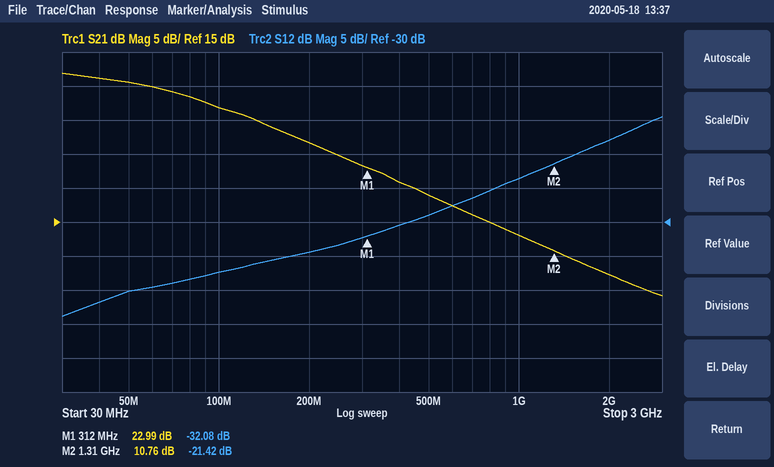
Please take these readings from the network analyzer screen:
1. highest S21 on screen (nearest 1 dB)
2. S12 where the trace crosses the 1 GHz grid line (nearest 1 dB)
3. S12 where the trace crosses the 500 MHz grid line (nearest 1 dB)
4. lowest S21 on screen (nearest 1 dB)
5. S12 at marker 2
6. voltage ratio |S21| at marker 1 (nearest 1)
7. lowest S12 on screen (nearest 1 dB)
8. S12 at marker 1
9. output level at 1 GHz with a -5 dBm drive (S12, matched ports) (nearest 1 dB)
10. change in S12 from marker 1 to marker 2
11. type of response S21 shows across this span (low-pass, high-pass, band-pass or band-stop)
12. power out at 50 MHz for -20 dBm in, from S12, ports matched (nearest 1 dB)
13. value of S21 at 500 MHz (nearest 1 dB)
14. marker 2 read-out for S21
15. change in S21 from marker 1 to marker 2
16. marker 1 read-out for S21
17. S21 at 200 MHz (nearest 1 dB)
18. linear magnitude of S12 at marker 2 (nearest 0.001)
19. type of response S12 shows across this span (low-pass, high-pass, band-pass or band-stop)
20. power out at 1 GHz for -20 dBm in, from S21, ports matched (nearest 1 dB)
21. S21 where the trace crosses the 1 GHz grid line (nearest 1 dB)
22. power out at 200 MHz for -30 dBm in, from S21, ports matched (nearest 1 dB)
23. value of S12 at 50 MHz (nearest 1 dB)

37 dB
-24 dB
-29 dB
4 dB
-21.42 dB
14
-44 dB
-32.08 dB
-29 dBm
10.66 dB
low-pass
-60 dBm
19 dB
10.76 dB
-12.23 dB
22.99 dB
27 dB
0.085
high-pass
-7 dBm
13 dB
-3 dBm
-40 dB
